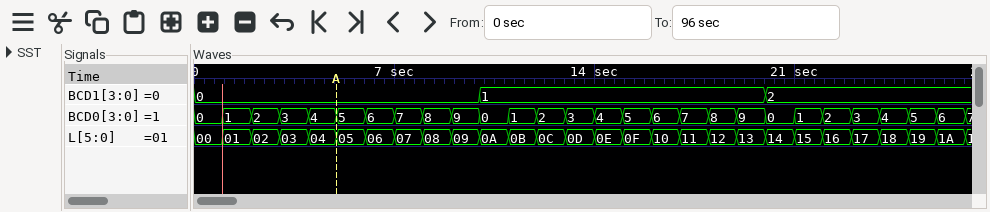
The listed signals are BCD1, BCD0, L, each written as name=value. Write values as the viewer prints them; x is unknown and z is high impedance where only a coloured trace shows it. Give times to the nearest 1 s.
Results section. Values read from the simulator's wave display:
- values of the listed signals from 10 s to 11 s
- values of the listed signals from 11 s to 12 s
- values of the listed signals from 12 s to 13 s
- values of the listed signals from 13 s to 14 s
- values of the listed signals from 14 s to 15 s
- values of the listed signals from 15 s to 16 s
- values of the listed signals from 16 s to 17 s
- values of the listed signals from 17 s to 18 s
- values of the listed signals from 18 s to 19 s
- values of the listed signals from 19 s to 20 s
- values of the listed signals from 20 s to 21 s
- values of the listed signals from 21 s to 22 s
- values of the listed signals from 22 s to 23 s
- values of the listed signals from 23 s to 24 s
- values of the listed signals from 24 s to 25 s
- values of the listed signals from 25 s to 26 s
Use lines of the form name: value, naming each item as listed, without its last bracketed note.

values of the listed signals from 10 s to 11 s: BCD1=1, BCD0=0, L=0A
values of the listed signals from 11 s to 12 s: BCD1=1, BCD0=1, L=0B
values of the listed signals from 12 s to 13 s: BCD1=1, BCD0=2, L=0C
values of the listed signals from 13 s to 14 s: BCD1=1, BCD0=3, L=0D
values of the listed signals from 14 s to 15 s: BCD1=1, BCD0=4, L=0E
values of the listed signals from 15 s to 16 s: BCD1=1, BCD0=5, L=0F
values of the listed signals from 16 s to 17 s: BCD1=1, BCD0=6, L=10
values of the listed signals from 17 s to 18 s: BCD1=1, BCD0=7, L=11
values of the listed signals from 18 s to 19 s: BCD1=1, BCD0=8, L=12
values of the listed signals from 19 s to 20 s: BCD1=1, BCD0=9, L=13
values of the listed signals from 20 s to 21 s: BCD1=2, BCD0=0, L=14
values of the listed signals from 21 s to 22 s: BCD1=2, BCD0=1, L=15
values of the listed signals from 22 s to 23 s: BCD1=2, BCD0=2, L=16
values of the listed signals from 23 s to 24 s: BCD1=2, BCD0=3, L=17
values of the listed signals from 24 s to 25 s: BCD1=2, BCD0=4, L=18
values of the listed signals from 25 s to 26 s: BCD1=2, BCD0=5, L=19
